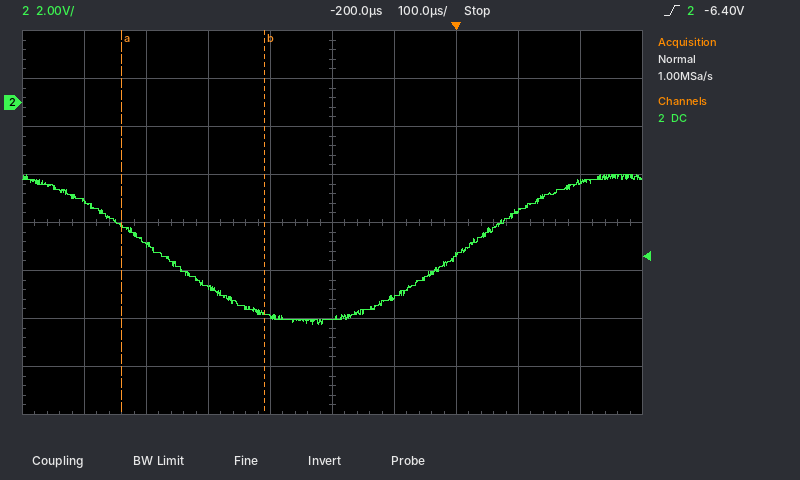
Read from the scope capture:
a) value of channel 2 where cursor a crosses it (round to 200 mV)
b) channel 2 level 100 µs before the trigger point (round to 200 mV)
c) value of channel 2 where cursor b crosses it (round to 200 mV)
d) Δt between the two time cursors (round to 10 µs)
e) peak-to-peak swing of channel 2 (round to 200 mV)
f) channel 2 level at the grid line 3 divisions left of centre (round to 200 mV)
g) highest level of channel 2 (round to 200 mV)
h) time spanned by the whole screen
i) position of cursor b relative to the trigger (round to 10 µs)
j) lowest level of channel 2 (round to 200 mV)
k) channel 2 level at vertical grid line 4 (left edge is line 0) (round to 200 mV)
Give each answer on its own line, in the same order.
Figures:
-5.2 V
-8.2 V
-8.8 V
230 µs
6.2 V
-6.0 V
-3.0 V
1 ms
-310 µs
-9.2 V
-9.0 V
